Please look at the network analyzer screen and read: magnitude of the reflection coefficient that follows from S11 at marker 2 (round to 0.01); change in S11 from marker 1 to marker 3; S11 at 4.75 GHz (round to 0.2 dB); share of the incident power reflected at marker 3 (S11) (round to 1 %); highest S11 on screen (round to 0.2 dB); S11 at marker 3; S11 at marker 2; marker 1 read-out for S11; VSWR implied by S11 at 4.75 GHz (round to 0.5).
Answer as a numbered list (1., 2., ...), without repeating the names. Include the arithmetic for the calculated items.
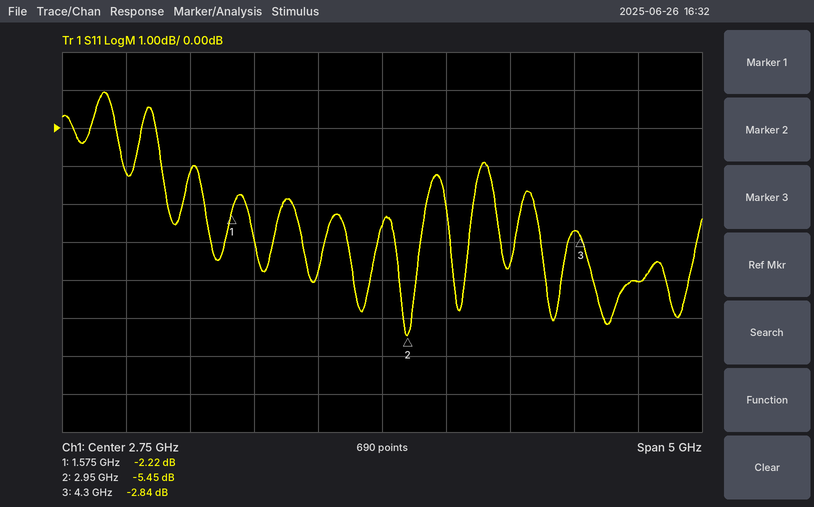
1. 10^(-5.45/20) ≈ 0.53
2. -2.84 − (-2.22) = -0.62 dB
3. -4.0 dB
4. 10^(-2.84/10) ≈ 52 %
5. 1.0 dB
6. -2.84 dB
7. -5.45 dB
8. -2.22 dB
9. |Γ| = 10^(-4/20) = 0.6310; VSWR = (1 + 0.6310)/(1 − 0.6310) ≈ 4.42, so 4.5 to the nearest 0.5
